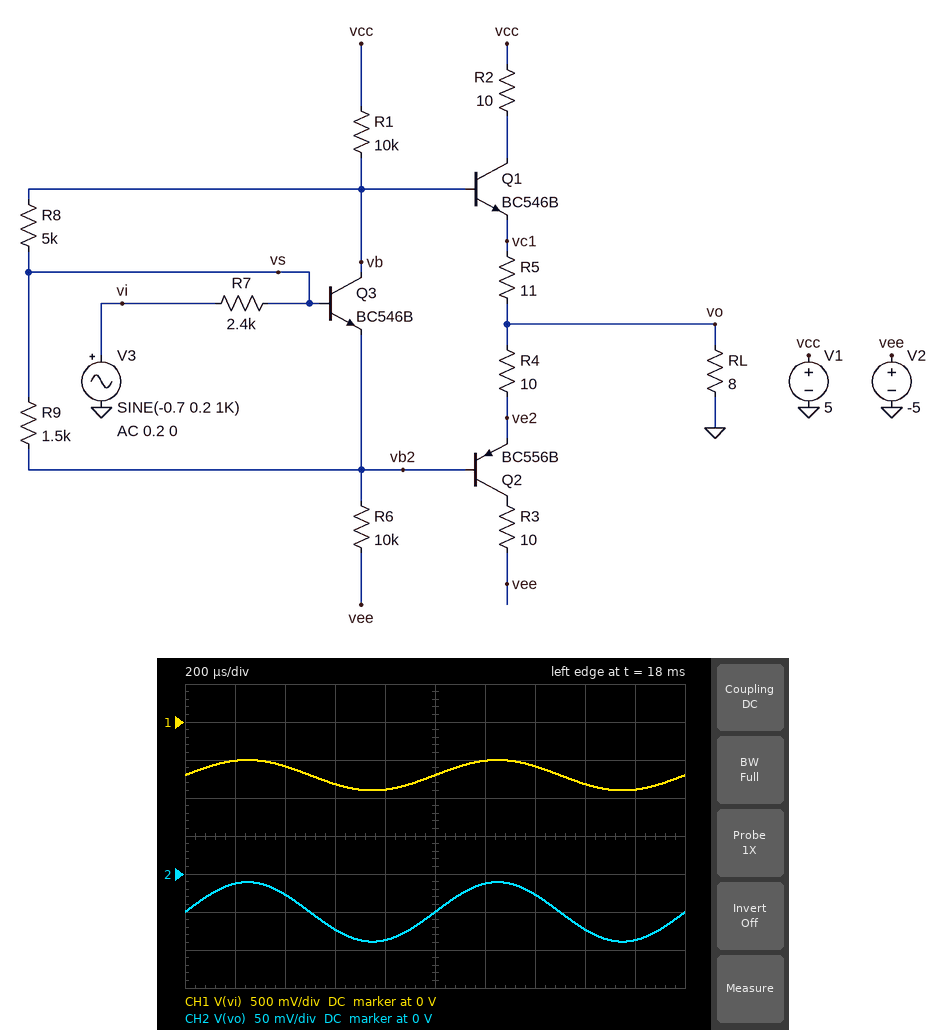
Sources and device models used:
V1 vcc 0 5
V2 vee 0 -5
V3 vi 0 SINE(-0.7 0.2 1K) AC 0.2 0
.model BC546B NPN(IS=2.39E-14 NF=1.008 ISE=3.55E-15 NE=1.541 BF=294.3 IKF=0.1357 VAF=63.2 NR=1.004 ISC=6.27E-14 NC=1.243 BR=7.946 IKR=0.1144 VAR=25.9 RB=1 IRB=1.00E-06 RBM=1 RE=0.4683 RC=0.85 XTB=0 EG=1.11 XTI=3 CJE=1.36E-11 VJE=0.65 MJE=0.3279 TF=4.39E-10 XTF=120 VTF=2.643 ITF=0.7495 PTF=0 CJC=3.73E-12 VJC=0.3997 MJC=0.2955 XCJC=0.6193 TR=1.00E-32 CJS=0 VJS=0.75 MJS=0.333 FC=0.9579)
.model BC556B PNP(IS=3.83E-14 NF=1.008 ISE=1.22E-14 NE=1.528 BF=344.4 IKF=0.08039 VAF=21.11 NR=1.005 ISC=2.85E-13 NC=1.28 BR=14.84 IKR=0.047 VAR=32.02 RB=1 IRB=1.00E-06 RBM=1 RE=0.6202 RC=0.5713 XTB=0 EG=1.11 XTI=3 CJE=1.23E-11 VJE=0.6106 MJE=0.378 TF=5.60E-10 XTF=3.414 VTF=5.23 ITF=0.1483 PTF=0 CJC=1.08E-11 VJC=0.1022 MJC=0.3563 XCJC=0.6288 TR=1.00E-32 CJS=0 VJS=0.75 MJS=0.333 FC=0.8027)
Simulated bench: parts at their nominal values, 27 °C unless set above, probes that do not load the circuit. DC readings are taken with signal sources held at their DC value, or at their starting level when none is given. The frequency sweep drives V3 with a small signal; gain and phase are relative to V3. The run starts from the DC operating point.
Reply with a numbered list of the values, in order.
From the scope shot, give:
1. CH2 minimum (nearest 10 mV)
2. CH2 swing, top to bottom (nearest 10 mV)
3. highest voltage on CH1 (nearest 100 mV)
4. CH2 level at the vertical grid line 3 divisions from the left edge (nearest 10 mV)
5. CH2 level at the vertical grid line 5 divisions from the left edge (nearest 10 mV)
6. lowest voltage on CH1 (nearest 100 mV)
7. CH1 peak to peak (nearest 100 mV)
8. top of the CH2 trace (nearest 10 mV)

1. -90 mV
2. 80 mV
3. -500 mV
4. -70 mV
5. -50 mV
6. -900 mV
7. 400 mV
8. -10 mV
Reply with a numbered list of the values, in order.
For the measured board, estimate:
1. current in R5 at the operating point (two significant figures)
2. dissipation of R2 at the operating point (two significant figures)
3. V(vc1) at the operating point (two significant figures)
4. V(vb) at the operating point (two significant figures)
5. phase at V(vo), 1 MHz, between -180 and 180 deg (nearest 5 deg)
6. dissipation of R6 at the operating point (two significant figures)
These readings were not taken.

1. 23 mA
2. 5.4 mW
3. 210 mV
4. 940 mV
5. -20 deg
6. 1.5 mW
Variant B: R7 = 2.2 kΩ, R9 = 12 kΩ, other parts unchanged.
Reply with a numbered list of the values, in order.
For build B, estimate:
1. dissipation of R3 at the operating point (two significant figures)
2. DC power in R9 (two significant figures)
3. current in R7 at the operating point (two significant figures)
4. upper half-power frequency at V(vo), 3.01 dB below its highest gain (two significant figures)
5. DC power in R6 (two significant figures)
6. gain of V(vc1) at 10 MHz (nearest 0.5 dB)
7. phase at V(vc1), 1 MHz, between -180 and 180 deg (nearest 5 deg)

1. 3.4 mW
2. 31 µW
3. 120 µA
4. 14 MHz
5. 1.6 mW
6. -13.0 dB
7. -10 deg
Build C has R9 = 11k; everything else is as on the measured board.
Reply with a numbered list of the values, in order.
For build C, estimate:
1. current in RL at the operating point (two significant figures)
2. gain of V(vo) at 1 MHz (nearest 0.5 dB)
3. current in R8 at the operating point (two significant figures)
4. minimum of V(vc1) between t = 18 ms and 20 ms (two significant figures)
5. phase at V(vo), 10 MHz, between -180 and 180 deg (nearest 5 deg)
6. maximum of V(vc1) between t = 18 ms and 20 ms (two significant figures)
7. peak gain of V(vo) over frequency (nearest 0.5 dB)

1. 18 mA
2. -13.0 dB
3. 170 µA
4. -180 mV
5. -60 deg
6. -94 mV
7. -12.5 dB
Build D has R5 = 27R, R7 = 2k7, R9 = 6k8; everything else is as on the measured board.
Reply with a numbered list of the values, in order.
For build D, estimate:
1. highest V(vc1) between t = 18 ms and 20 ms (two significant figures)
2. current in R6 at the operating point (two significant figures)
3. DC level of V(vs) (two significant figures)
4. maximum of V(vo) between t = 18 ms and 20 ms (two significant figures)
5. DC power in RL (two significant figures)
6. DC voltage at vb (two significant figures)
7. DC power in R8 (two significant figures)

1. -87 mV
2. 400 µA
3. -430 mV
4. -93 mV
5. 2.3 mW
6. 530 mV
7. 180 µW
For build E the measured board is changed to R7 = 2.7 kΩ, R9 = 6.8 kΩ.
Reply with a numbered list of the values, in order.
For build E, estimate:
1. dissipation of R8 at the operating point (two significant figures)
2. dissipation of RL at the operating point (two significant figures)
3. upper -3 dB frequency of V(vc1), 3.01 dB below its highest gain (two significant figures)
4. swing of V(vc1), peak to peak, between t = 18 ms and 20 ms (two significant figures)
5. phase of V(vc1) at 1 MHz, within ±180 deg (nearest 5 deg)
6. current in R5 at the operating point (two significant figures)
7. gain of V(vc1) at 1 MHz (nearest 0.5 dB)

1. 180 µW
2. 2.3 mW
3. 1.2 MHz
4. 41 mV
5. -45 deg
6. 1.3 mA
7. -22.0 dB
